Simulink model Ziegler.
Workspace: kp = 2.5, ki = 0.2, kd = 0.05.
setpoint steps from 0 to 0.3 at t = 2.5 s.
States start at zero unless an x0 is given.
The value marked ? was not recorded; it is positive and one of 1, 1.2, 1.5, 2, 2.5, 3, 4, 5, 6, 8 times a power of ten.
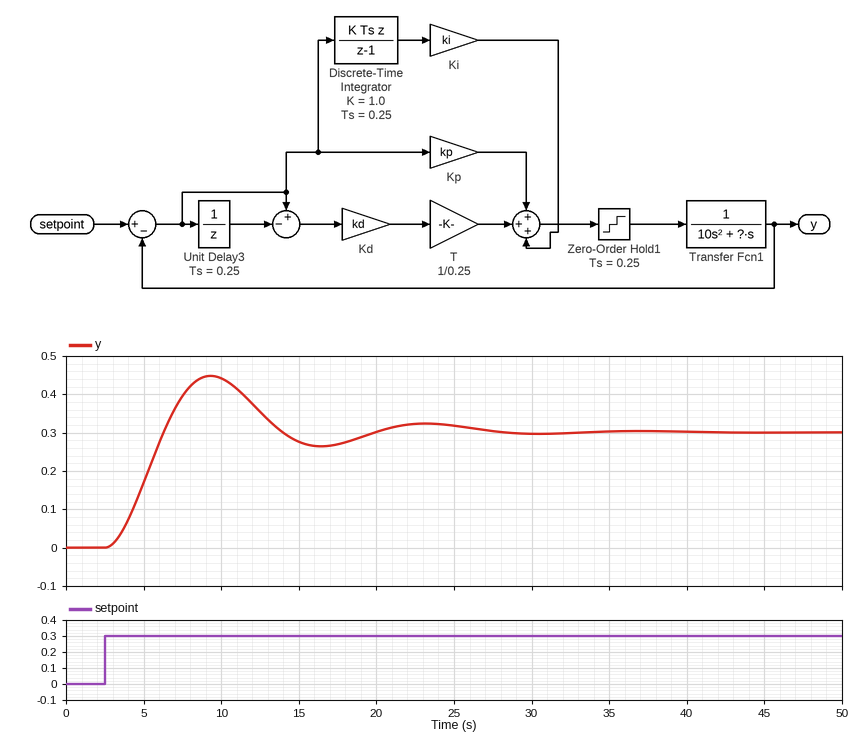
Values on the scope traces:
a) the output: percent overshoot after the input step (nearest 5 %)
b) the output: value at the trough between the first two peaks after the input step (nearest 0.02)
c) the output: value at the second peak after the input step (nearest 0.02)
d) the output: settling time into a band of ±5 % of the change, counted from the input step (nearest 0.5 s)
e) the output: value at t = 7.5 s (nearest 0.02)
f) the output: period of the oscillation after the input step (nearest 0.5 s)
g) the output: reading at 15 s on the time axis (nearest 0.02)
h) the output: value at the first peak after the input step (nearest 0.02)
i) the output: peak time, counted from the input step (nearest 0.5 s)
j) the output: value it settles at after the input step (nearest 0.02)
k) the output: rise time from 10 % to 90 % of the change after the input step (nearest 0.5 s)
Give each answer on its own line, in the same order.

50 %
0.26
0.32
23.0 s
0.40
14.0 s
0.28
0.44
7.0 s
0.30
2.5 s
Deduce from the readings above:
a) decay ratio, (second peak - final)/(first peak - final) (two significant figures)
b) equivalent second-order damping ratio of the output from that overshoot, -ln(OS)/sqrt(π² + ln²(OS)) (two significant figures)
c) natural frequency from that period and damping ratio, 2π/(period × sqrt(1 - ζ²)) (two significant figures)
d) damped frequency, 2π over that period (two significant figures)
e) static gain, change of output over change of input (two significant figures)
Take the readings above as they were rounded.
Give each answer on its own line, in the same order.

0.14
0.22
0.46 rad/s
0.45 rad/s
1.0
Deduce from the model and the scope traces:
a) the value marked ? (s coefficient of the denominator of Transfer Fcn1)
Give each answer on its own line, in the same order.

4
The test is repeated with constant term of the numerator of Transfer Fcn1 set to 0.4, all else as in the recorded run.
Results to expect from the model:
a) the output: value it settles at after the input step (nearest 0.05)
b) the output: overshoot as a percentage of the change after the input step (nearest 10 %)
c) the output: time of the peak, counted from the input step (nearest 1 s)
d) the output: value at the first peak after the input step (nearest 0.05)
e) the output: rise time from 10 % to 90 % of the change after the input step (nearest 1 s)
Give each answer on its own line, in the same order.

0.30
40 %
12 s
0.40
5 s
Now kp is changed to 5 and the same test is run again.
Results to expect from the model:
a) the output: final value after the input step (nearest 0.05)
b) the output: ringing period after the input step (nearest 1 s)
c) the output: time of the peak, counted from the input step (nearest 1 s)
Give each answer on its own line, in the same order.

0.30
9 s
5 s
